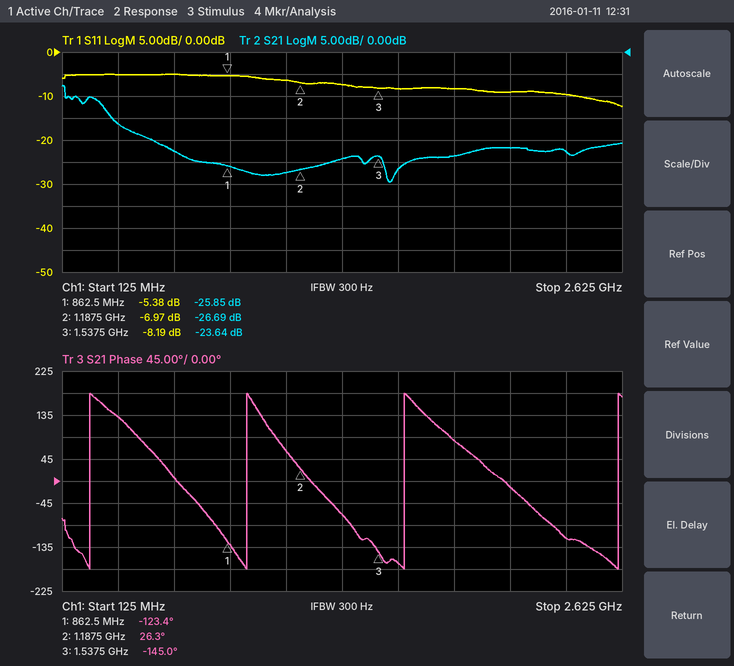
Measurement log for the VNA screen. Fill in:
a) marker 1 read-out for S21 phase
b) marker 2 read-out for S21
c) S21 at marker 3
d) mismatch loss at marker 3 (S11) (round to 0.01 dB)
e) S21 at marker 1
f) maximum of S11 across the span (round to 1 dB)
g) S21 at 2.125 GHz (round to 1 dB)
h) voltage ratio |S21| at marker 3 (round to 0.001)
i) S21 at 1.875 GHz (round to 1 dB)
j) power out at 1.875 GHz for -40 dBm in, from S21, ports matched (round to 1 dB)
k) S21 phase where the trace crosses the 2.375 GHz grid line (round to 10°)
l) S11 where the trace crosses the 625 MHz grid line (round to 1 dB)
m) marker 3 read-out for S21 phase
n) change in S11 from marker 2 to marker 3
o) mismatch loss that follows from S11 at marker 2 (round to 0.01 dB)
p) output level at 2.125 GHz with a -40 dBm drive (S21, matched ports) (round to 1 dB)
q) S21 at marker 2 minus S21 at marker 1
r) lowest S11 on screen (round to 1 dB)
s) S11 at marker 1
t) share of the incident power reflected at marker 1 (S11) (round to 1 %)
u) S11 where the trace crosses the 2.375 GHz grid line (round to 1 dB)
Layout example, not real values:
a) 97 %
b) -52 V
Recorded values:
a) -123.4°
b) -26.69 dB
c) -23.64 dB
d) 0.71 dB
e) -25.85 dB
f) -5 dB
g) -22 dB
h) 0.066
i) -24 dB
j) -64 dBm
k) -120°
l) -5 dB
m) -145.0°
n) -1.22 dB
o) 0.97 dB
p) -62 dBm
q) -0.84 dB
r) -12 dB
s) -5.38 dB
t) 29 %
u) -10 dB
